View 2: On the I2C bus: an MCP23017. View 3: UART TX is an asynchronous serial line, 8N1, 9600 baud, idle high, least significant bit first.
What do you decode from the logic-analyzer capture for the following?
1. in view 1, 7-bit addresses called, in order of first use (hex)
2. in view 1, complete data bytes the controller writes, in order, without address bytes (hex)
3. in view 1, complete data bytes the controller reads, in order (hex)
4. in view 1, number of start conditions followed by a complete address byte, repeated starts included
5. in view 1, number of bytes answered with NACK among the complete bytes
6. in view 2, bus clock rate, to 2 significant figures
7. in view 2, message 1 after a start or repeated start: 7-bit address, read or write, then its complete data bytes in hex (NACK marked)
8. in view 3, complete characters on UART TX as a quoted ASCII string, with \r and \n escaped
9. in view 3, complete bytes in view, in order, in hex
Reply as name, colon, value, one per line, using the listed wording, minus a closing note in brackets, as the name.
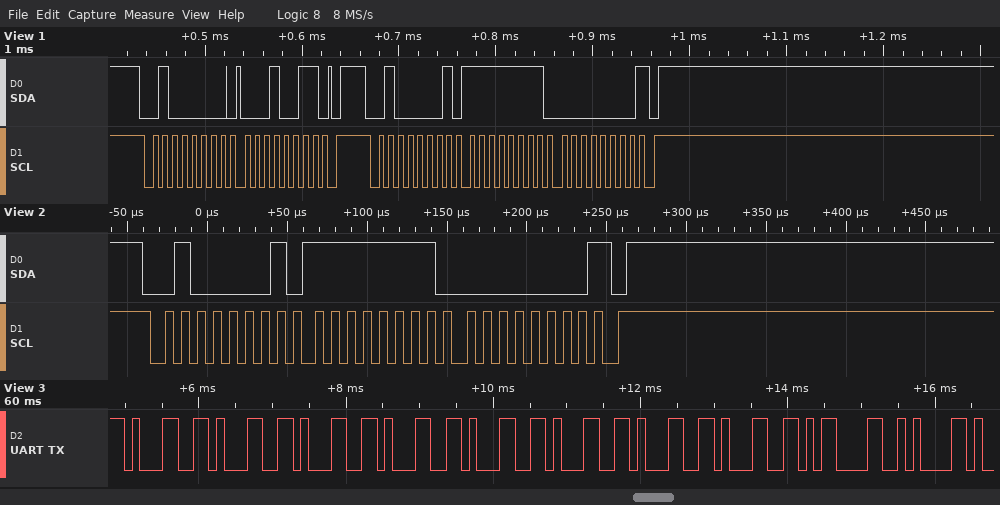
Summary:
in view 1, 7-bit addresses called, in order of first use: 0x20
in view 1, complete data bytes the controller writes, in order, without address bytes: 13
in view 1, complete data bytes the controller reads, in order: FF 00
in view 1, number of start conditions followed by a complete address byte, repeated starts included: 2
in view 1, number of bytes answered with NACK among the complete bytes: 1
in view 2, bus clock rate, to 2 significant figures: 100 kHz
in view 2, message 1 after a start or repeated start: 7-bit address, read or write, then its complete data bytes in hex: 0x20 read: FF 00 NACK
in view 3, complete characters on UART TX as a quoted ASCII string, with \r and \n escaped: "11111111\r\n"
in view 3, complete bytes in view, in order, in hex: 31 31 31 31 31 31 31 31 0D 0A
